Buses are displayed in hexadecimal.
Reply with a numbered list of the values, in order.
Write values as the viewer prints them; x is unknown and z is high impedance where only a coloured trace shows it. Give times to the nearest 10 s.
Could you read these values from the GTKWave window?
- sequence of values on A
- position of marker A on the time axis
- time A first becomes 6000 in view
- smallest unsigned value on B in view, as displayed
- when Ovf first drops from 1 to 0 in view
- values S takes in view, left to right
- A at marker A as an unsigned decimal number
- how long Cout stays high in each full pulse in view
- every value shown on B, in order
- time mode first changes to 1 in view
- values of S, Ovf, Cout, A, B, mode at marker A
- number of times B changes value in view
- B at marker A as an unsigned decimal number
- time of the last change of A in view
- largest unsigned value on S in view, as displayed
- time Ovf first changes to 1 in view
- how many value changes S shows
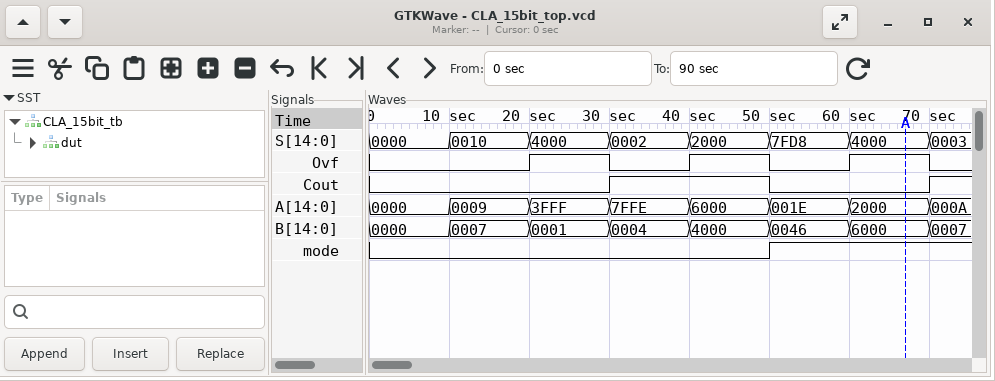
1. 0000, 0009, 3FFF, 7FFE, 6000, 001E, 2000, 000A
2. 70 s
3. 40 s
4. 0000
5. 30 s
6. 0000, 0010, 4000, 0002, 2000, 7FD8, 4000, 0003
7. 8192
8. 20 s
9. 0000, 0007, 0001, 0004, 4000, 0046, 6000, 0007
10. 50 s
11. S=4000, Ovf=1, Cout=0, A=2000, B=6000, mode=1
12. 7
13. 24576
14. 70 s
15. 7FD8
16. 20 s
17. 7
